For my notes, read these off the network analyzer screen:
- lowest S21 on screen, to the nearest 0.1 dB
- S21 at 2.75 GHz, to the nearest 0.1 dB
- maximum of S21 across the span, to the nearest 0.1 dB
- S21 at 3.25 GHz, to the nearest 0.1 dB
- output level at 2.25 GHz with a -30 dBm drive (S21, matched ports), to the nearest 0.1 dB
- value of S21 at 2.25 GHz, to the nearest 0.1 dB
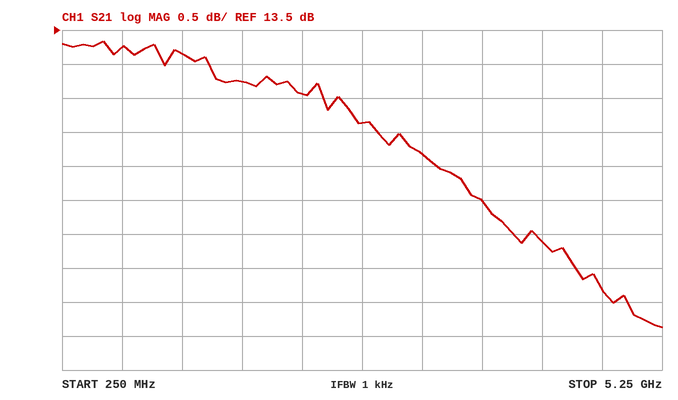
9.1 dB
12.1 dB
13.3 dB
11.7 dB
-17.4 dBm
12.6 dB
